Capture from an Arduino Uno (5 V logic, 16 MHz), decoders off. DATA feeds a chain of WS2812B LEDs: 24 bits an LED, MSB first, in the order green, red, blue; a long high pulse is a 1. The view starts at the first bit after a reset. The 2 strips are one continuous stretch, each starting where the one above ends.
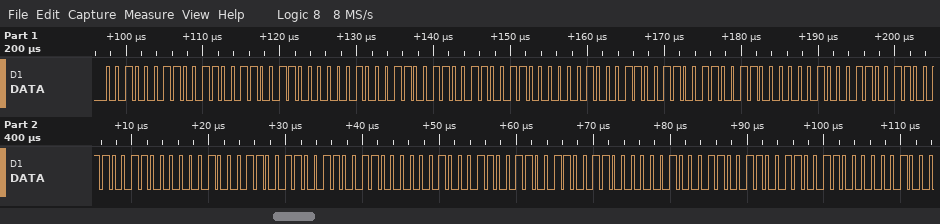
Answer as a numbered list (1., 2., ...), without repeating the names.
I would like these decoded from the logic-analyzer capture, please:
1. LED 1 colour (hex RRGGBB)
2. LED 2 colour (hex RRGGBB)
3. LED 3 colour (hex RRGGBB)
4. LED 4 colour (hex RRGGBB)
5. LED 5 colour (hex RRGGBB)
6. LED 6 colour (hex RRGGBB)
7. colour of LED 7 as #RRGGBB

1. #332330
2. #332330
3. #332330
4. #332330
5. #332330
6. #332330
7. #332330
